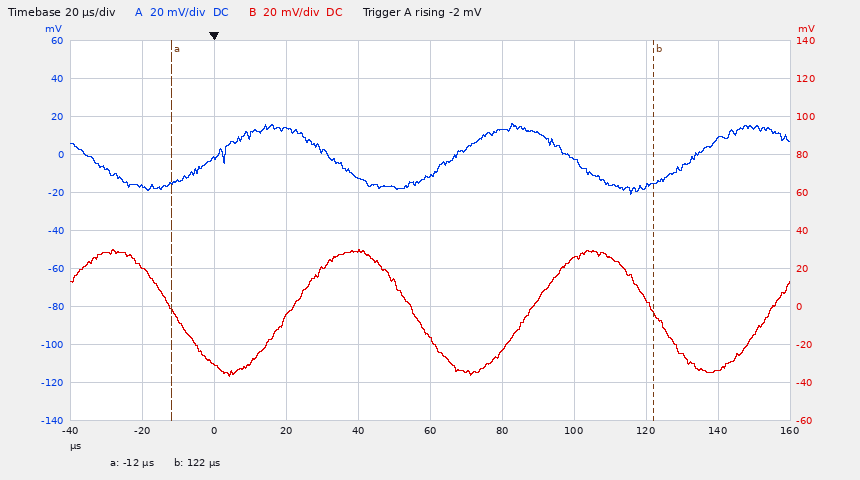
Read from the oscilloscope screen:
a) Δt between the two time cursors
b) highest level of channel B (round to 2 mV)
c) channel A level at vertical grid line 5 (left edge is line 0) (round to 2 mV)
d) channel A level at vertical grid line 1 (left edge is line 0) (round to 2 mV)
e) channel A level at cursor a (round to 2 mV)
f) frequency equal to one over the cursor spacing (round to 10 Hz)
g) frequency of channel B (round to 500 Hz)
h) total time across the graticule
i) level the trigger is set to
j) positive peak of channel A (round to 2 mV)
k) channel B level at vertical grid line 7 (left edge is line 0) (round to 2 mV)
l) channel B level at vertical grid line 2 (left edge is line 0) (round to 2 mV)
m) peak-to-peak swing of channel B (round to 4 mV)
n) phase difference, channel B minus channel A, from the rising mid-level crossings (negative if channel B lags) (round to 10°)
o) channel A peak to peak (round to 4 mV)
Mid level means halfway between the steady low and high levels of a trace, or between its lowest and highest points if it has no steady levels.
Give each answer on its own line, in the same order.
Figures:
134 µs
30 mV
-12 mV
-16 mV
-16 mV
7.46 kHz
15.0 kHz
200 µs
-2 mV
16 mV
26 mV
-30 mV
68 mV
-110°
36 mV
